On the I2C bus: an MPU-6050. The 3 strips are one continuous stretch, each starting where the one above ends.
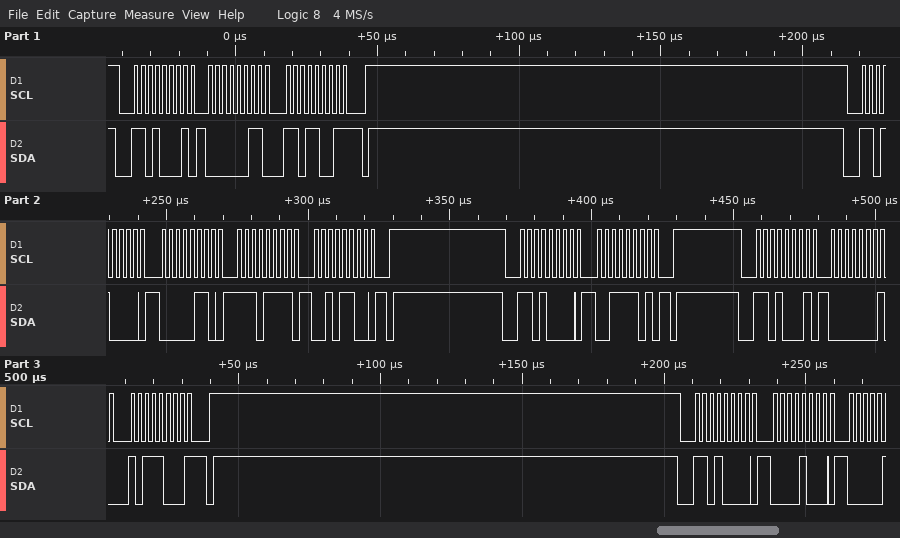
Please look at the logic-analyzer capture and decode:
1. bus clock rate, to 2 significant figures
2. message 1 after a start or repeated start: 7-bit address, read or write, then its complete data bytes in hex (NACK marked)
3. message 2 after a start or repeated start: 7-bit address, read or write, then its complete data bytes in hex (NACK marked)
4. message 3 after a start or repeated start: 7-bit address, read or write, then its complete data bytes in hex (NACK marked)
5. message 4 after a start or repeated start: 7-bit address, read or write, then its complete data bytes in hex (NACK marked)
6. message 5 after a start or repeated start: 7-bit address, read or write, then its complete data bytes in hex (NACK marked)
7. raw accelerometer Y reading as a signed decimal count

400 kHz
0x68 read: 03 D9 NACK
0x68 write: 06 EF 2C
0x68 write: 3D
0x68 read: 01 B8 NACK
0x68 write: 08
440
